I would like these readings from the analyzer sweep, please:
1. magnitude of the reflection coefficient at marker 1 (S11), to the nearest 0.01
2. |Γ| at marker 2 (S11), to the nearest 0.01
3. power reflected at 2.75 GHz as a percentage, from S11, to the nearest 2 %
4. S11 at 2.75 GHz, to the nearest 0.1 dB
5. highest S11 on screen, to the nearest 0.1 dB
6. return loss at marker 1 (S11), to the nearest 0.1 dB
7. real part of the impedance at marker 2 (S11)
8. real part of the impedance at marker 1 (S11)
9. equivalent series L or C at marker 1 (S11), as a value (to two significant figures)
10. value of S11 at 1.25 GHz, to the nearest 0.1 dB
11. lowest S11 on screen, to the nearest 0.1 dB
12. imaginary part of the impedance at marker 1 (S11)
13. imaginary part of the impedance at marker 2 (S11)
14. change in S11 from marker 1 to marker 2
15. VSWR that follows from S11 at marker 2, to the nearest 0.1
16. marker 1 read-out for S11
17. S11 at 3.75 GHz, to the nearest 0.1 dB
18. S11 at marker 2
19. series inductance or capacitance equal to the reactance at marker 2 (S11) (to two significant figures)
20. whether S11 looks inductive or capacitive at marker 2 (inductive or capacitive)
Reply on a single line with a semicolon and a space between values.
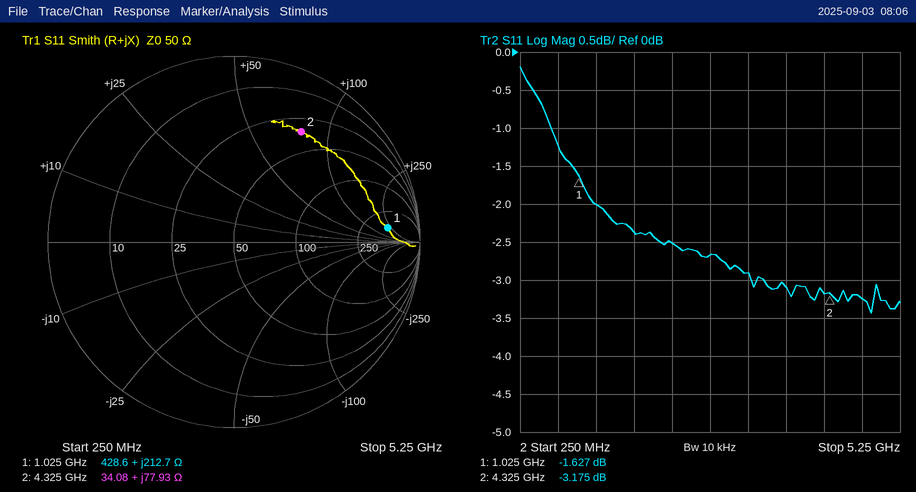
0.83; 0.69; 54 %; -2.7 dB; -0.2 dB; 1.6 dB; 34.08 Ω; 428.6 Ω; 33 nH; -2.0 dB; -3.4 dB; +212.7 Ω; +77.93 Ω; -1.548 dB; 5.5; -1.627 dB; -3.1 dB; -3.175 dB; 2.9 nH; inductive
